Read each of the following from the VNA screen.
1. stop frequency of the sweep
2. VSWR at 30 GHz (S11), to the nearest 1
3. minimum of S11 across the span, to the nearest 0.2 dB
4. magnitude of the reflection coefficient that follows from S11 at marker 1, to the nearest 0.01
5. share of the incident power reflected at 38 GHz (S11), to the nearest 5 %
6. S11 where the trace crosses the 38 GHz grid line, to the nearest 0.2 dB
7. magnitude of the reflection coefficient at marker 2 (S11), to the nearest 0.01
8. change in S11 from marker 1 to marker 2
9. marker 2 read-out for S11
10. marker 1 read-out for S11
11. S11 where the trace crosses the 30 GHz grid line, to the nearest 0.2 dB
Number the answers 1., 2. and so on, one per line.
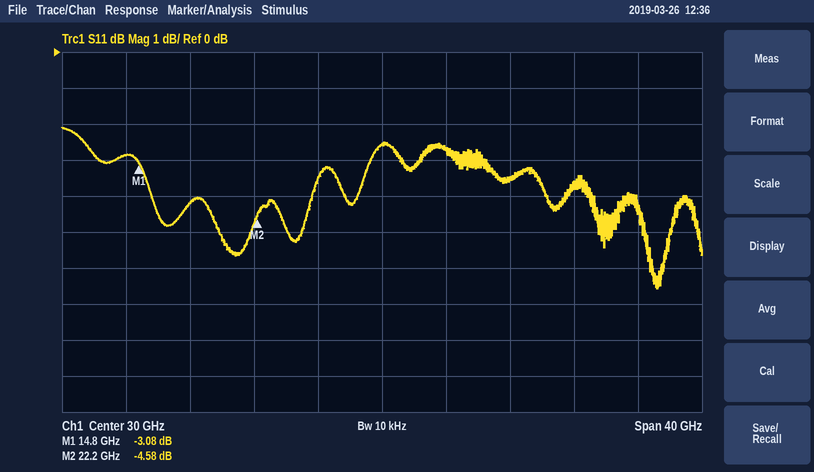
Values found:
1. 50 GHz
2. 7
3. -6.6 dB
4. 0.70
5. 45 %
6. -3.6 dB
7. 0.59
8. -1.50 dB
9. -4.58 dB
10. -3.08 dB
11. -2.6 dB
